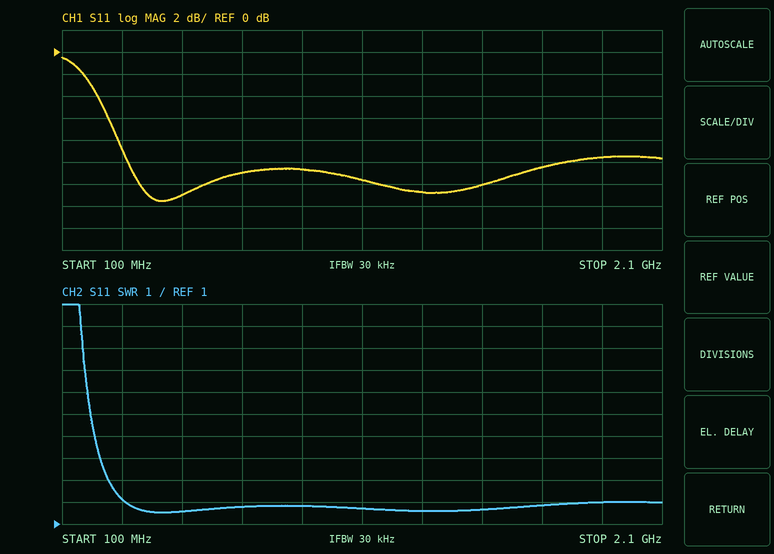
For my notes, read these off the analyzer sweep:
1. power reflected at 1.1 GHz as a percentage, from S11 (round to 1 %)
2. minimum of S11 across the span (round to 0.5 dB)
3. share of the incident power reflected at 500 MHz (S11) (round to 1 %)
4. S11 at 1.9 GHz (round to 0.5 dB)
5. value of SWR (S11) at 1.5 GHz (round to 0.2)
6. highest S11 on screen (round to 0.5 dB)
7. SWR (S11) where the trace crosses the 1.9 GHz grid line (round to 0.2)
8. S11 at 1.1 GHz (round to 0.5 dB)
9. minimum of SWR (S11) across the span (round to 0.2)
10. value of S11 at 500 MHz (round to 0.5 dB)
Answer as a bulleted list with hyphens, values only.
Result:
- 7 %
- -13.5 dB
- 5 %
- -9.5 dB
- 1.6
- -0.5 dB
- 2.0
- -11.5 dB
- 1.6
- -13.0 dB
